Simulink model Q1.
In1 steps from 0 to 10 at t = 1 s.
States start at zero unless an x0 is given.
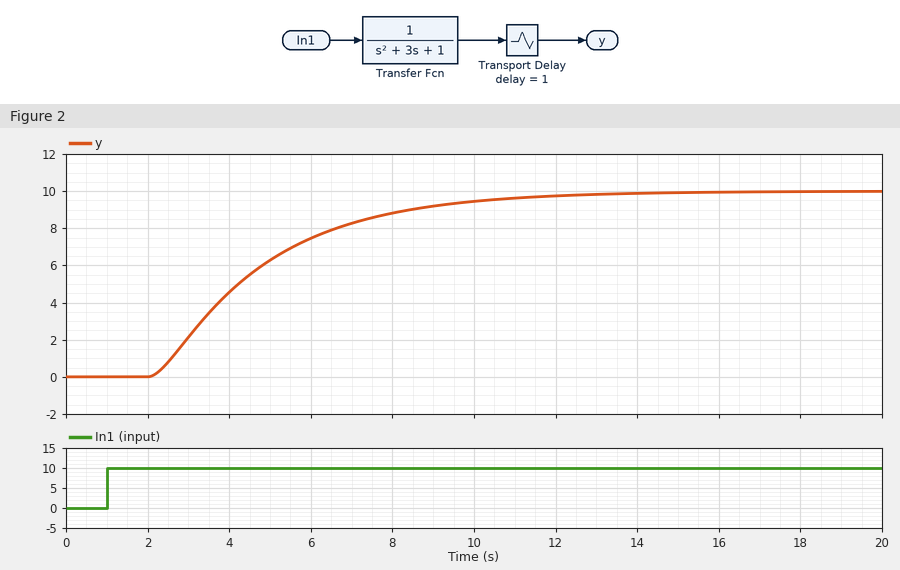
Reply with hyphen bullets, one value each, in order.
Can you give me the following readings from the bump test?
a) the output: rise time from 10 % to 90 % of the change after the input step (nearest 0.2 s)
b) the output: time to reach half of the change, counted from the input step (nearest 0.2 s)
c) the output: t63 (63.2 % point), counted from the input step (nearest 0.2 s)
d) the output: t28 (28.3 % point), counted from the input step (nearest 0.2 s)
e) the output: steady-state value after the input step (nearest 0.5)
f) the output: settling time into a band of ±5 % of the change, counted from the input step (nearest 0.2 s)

- 5.8 s
- 3.2 s
- 4.0 s
- 2.2 s
- 10.0
- 9.2 s
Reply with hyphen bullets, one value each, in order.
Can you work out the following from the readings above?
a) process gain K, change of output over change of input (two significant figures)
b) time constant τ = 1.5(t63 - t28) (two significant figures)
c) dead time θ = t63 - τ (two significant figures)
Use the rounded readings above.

- 1.0
- 2.7 s
- 1.3 s
